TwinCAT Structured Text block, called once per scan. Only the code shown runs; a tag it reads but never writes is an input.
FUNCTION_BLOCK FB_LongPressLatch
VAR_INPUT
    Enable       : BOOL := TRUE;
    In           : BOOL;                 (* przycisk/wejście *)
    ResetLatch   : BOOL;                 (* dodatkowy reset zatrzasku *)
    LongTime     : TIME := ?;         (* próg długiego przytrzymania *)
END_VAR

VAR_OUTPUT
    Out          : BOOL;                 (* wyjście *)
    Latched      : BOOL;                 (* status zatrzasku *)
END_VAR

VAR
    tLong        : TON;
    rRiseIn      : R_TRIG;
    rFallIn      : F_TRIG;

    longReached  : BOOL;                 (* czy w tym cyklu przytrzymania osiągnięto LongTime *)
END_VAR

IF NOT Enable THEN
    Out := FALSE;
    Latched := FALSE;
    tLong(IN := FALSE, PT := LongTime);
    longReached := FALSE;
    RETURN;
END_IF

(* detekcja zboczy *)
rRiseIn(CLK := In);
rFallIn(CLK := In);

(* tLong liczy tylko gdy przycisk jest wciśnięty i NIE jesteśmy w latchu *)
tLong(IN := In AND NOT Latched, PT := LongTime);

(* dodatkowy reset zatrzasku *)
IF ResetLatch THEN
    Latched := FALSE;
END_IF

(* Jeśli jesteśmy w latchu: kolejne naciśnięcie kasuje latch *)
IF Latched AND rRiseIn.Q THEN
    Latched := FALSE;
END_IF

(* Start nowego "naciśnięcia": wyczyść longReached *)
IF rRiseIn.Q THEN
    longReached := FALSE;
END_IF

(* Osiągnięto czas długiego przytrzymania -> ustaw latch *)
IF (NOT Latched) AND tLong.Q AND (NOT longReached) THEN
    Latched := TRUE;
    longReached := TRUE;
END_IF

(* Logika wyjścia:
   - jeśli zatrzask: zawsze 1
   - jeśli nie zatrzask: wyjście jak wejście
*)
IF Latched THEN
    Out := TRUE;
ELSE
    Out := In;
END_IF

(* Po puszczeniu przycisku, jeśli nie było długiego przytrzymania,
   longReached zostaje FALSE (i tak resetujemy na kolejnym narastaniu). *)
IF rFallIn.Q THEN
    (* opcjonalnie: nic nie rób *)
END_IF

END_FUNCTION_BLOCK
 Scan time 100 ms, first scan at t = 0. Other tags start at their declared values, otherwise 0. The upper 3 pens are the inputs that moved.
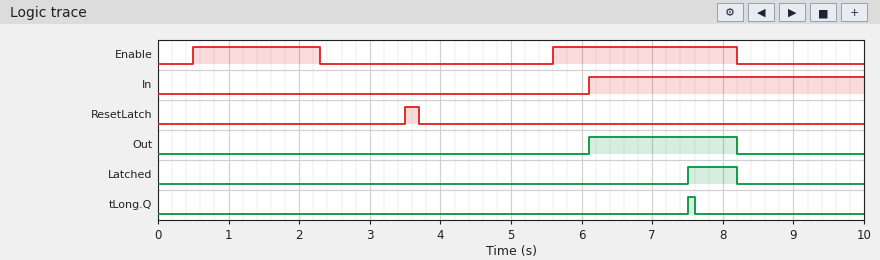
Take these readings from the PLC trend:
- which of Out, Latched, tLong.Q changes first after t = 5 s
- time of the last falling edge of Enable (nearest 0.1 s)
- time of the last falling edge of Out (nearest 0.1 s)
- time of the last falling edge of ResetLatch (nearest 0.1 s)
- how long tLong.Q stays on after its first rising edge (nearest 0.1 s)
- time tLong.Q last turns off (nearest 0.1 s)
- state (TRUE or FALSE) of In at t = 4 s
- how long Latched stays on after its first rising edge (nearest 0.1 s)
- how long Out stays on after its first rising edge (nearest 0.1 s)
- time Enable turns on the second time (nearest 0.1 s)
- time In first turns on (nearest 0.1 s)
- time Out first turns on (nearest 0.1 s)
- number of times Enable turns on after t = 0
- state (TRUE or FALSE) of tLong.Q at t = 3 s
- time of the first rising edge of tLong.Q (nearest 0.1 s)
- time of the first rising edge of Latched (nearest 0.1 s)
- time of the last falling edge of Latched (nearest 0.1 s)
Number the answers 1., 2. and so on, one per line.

1. Out
2. 8.2 s
3. 8.2 s
4. 3.7 s
5. 0.1 s
6. 7.6 s
7. FALSE
8. 0.7 s
9. 2.1 s
10. 5.6 s
11. 6.1 s
12. 6.1 s
13. 2
14. FALSE
15. 7.5 s
16. 7.5 s
17. 8.2 s
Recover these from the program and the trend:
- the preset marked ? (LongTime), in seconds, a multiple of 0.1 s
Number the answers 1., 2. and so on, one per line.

1. 1.4 s
